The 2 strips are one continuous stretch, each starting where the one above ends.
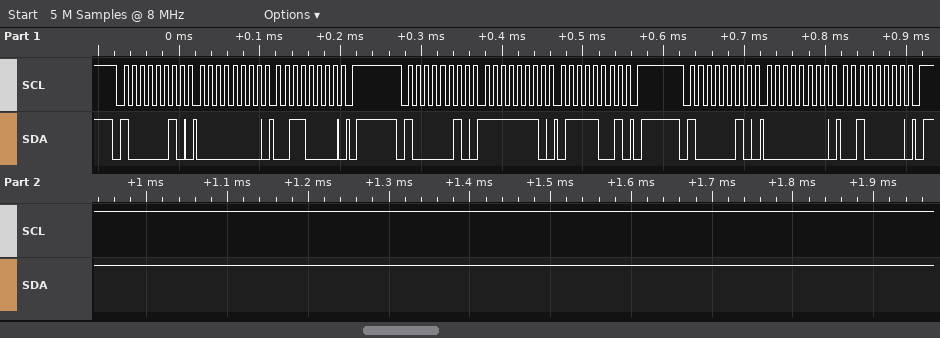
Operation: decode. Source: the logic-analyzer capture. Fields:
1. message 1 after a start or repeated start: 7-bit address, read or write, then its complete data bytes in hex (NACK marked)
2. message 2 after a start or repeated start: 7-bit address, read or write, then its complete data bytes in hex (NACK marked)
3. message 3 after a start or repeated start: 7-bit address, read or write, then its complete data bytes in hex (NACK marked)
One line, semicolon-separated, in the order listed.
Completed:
0x41 write: 00 30; 0x41 write: FE 79; 0x41 write: 00 20
